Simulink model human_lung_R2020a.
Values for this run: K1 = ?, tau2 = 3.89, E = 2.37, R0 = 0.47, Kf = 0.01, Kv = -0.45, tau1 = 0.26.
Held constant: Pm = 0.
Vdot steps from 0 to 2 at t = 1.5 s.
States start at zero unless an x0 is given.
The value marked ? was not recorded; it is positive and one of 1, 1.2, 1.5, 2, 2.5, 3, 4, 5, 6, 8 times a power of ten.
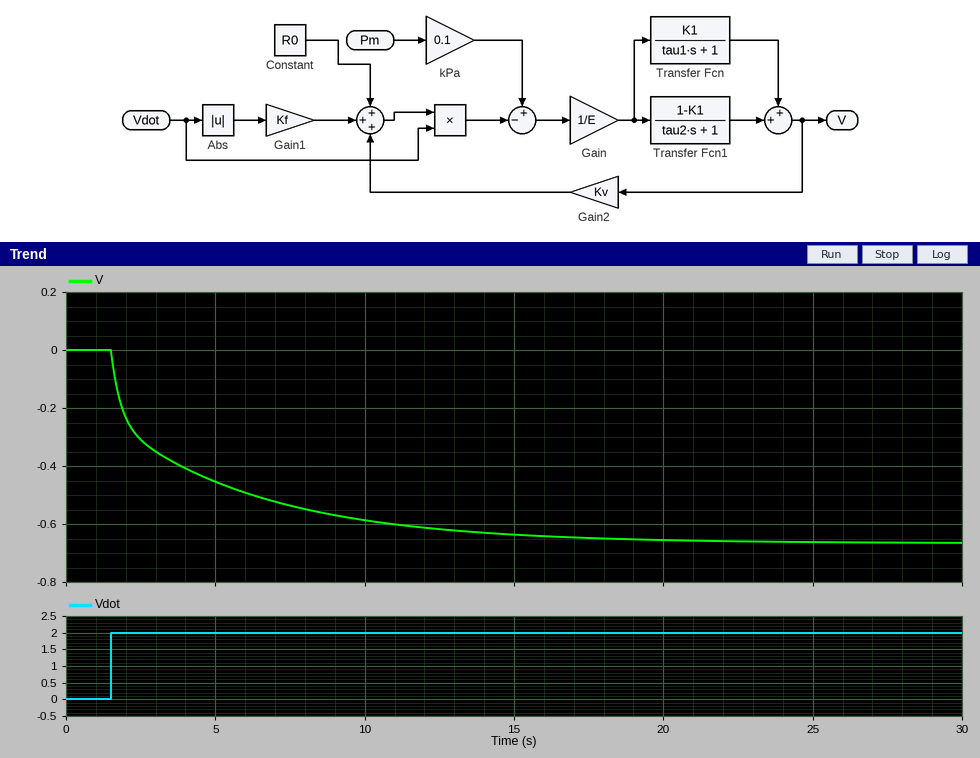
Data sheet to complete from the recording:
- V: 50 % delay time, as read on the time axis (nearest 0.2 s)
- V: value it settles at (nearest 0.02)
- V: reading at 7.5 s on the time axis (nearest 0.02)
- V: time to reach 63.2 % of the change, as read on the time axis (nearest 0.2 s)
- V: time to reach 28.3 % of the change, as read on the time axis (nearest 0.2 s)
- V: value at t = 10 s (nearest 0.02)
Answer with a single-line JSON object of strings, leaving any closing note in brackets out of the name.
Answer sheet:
{"V: 50 % delay time, as read on the time axis": "2.8 s", "V: value it settles at": "-0.66", "V: reading at 7.5 s on the time axis": "-0.54", "V: time to reach 63.2 % of the change, as read on the time axis": "4.2 s", "V: time to reach 28.3 % of the change, as read on the time axis": "1.8 s", "V: value at t = 10 s": "-0.58"}
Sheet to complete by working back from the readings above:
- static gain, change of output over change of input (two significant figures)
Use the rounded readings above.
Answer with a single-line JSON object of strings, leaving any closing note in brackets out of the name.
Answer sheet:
{"static gain, change of output over change of input": "-0.33"}
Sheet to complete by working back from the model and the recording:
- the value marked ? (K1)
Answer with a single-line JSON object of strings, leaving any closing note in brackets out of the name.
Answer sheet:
{"the value marked ?": "0.5"}
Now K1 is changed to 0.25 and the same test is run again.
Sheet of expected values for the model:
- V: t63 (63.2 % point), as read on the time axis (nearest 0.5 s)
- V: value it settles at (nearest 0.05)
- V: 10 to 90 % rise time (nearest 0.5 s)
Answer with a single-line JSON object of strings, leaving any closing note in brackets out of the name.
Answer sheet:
{"V: t63 (63.2 % point), as read on the time axis": "6.0 s", "V: value it settles at": "-0.65", "V: 10 to 90 % rise time": "12.0 s"}
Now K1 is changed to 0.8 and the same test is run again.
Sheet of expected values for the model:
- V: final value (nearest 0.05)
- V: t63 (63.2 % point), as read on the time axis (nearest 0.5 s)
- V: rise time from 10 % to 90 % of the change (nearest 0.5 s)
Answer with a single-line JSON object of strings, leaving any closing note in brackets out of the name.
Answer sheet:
{"V: final value": "-0.65", "V: t63 (63.2 % point), as read on the time axis": "2.0 s", "V: rise time from 10 % to 90 % of the change": "5.0 s"}
